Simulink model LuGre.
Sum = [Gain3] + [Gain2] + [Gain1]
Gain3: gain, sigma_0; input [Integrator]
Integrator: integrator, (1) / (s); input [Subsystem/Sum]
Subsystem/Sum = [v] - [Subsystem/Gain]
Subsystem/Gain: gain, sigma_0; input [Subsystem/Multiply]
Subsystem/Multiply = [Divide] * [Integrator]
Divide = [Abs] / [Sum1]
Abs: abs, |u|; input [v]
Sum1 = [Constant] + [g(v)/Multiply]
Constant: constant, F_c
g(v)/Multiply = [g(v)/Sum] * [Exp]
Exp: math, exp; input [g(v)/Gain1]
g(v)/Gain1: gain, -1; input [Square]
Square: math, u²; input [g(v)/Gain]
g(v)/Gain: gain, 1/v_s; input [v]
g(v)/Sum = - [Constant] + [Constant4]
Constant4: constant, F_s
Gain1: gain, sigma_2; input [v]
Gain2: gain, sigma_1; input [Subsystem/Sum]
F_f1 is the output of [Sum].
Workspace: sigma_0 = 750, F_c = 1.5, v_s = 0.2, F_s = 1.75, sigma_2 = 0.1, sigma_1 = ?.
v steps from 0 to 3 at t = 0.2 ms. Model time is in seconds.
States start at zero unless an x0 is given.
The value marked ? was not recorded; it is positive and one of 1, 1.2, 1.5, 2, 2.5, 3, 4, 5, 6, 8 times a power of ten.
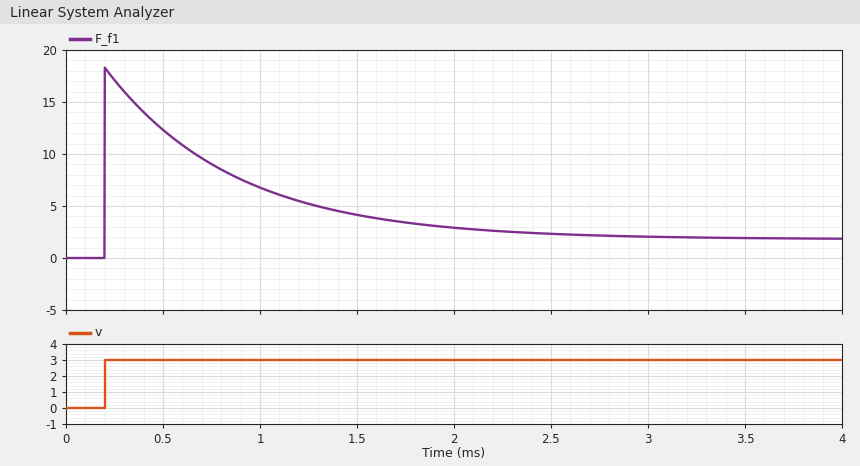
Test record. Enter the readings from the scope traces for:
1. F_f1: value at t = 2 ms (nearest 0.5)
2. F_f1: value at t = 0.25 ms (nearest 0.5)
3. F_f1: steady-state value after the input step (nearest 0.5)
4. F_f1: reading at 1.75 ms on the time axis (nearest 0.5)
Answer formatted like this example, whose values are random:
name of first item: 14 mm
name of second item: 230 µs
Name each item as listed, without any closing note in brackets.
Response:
F_f1: value at t = 2 ms: 3.0
F_f1: value at t = 0.25 ms: 17.0
F_f1: steady-state value after the input step: 2.0
F_f1: reading at 1.75 ms on the time axis: 3.5
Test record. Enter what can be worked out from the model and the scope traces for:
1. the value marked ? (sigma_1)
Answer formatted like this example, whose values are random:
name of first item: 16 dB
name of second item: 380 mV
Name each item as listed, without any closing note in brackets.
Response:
the value marked ?: 6
